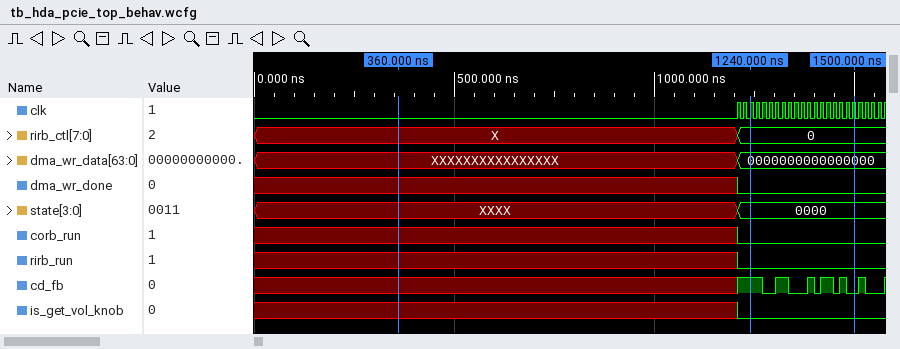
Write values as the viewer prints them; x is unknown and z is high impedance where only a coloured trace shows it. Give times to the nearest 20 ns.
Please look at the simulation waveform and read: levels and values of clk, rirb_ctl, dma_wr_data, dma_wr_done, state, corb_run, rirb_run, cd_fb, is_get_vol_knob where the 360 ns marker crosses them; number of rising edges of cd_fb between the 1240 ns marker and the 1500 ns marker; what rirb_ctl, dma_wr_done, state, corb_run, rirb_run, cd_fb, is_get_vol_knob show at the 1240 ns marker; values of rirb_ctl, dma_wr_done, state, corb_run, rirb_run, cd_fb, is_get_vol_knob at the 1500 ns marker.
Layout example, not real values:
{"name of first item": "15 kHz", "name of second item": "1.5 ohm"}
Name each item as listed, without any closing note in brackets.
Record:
{"levels and values of clk, rirb_ctl, dma_wr_data, dma_wr_done, state, corb_run, rirb_run, cd_fb, is_get_vol_knob where the 360 ns marker crosses them": "clk=0, rirb_ctl=X, dma_wr_data=XXXXXXXXXXXXXXXX, dma_wr_done=x, state=XXXX, corb_run=x, rirb_run=x, cd_fb=x, is_get_vol_knob=x", "number of rising edges of cd_fb between the 1240 ns marker and the 1500 ns marker": "4", "what rirb_ctl, dma_wr_done, state, corb_run, rirb_run, cd_fb, is_get_vol_knob show at the 1240 ns marker": "rirb_ctl=0, dma_wr_done=0, state=0000, corb_run=0, rirb_run=0, cd_fb=1, is_get_vol_knob=0", "values of rirb_ctl, dma_wr_done, state, corb_run, rirb_run, cd_fb, is_get_vol_knob at the 1500 ns marker": "rirb_ctl=0, dma_wr_done=0, state=0000, corb_run=0, rirb_run=0, cd_fb=0, is_get_vol_knob=0"}
